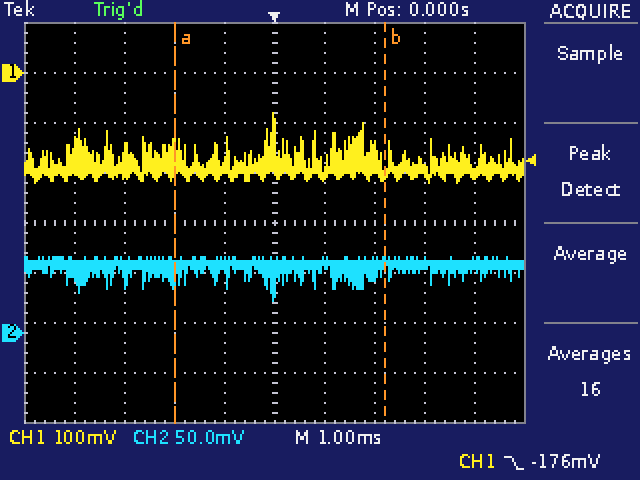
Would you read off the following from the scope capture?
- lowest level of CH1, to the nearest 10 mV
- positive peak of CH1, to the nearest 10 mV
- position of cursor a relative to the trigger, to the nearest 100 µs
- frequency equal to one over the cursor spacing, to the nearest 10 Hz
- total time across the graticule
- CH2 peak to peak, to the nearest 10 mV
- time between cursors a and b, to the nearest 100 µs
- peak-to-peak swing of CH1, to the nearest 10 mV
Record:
-220 mV
-80 mV
-2.0 ms
240 Hz
10 ms
40 mV
4.2 ms
140 mV
